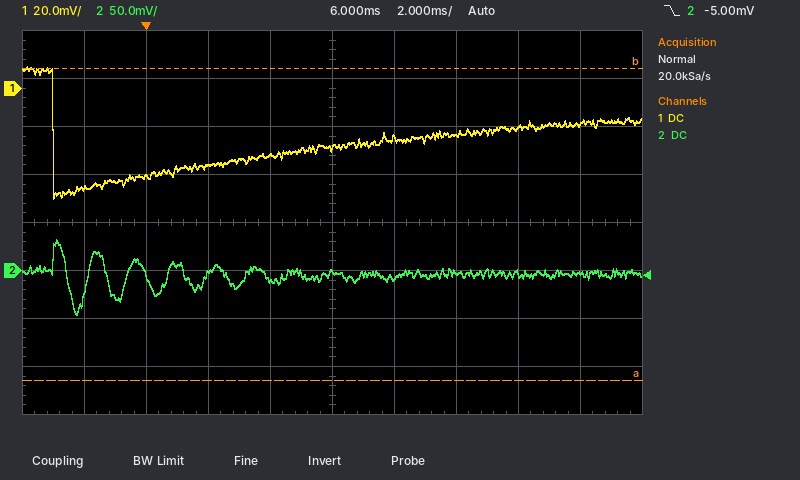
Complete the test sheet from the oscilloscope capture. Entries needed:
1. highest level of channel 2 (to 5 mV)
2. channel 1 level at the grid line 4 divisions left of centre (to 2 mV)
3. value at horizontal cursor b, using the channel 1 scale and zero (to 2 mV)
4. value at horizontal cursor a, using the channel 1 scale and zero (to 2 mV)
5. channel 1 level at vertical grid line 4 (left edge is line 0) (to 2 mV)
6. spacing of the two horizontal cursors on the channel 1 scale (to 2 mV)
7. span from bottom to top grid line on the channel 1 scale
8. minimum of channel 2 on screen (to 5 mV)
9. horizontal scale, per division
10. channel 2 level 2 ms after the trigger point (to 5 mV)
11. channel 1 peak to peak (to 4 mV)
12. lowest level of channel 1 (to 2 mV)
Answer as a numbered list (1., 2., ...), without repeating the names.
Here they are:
1. 30 mV
2. -42 mV
3. 8 mV
4. -122 mV
5. -28 mV
6. 130 mV
7. 160 mV
8. -45 mV
9. 2 ms
10. -5 mV
11. 56 mV
12. -46 mV
